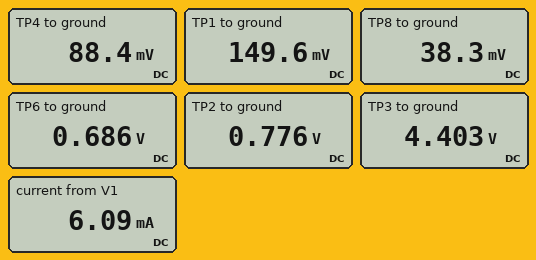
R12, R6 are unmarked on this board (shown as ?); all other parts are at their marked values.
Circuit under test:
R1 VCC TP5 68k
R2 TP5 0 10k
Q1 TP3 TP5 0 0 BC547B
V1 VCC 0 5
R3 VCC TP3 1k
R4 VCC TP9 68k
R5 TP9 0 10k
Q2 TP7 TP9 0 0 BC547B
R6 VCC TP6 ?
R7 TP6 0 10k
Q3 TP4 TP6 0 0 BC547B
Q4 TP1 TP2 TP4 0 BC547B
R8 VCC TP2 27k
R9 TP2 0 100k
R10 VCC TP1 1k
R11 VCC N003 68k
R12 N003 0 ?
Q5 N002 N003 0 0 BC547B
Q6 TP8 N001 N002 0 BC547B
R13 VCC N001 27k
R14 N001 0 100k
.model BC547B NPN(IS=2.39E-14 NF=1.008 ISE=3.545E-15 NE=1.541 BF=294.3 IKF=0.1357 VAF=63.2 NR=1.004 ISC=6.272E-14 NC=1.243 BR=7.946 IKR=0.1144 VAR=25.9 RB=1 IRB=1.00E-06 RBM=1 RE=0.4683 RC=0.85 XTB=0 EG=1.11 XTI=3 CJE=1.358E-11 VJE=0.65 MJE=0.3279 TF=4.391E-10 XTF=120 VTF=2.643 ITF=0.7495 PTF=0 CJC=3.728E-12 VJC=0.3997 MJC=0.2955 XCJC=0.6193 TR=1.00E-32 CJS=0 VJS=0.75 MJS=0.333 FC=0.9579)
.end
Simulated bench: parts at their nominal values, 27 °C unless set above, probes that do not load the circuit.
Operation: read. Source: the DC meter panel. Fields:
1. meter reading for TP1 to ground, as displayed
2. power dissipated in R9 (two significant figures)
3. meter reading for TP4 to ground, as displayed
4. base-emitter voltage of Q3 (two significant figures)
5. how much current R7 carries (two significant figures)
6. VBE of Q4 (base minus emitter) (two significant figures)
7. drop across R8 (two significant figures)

149.6 mV
6.0 µW
88.4 mV
690 mV
69 µA
690 mV
4.2 V
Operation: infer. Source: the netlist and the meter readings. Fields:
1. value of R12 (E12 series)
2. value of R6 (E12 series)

12 kΩ
33 kΩ
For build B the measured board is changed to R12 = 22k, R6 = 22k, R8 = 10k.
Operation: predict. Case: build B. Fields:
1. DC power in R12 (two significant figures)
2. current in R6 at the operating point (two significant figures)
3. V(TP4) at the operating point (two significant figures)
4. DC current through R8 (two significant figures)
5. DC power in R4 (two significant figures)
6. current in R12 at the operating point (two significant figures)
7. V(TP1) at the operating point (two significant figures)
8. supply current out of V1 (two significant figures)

17 µW
200 µA
68 mV
420 µA
290 µW
28 µA
110 mV
6.5 mA
